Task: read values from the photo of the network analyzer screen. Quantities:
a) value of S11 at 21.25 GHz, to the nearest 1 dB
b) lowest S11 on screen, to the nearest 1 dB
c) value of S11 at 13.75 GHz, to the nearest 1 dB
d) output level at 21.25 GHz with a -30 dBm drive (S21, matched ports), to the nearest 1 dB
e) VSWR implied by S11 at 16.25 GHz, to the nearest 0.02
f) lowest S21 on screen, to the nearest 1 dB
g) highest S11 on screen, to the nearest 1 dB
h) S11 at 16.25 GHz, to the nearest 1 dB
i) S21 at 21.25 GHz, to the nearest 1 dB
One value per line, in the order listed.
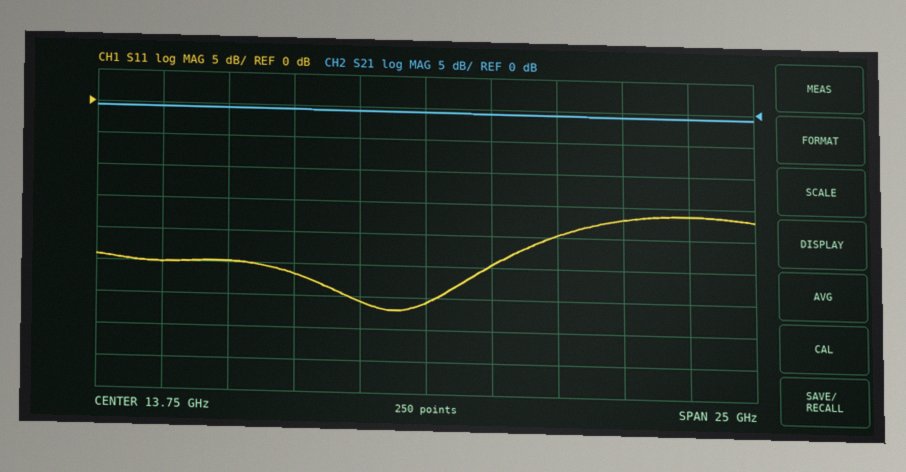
-17 dB
-32 dB
-31 dB
-31 dBm
1.12
-1 dB
-16 dB
-25 dB
-1 dB
